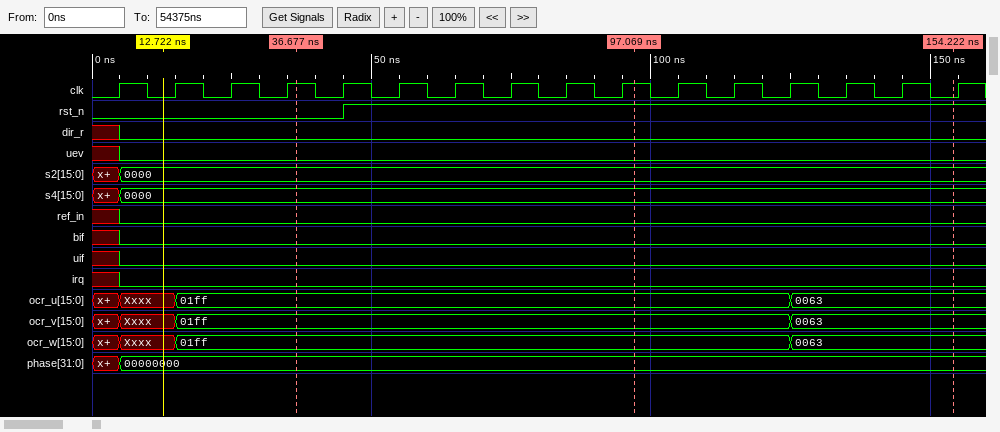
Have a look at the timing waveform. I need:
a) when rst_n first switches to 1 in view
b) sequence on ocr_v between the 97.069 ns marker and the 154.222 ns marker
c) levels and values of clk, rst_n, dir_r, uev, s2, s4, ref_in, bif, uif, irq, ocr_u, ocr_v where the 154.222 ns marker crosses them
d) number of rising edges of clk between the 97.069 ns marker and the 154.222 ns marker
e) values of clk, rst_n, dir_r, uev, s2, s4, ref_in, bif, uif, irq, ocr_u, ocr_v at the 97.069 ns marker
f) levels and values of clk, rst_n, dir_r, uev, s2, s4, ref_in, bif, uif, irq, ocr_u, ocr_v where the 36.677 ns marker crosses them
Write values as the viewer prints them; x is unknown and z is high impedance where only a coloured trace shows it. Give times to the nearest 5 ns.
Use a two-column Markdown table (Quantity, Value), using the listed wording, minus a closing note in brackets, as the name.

| Quantity | Value |
|---|---|
| when rst_n first switches to 1 in view | 45 ns |
| sequence on ocr_v between the 97.069 ns marker and the 154.222 ns marker | 01ff, 0063 |
| levels and values of clk, rst_n, dir_r, uev, s2, s4, ref_in, bif, uif, irq, ocr_u, ocr_v where the 154.222 ns marker crosses them | clk=0, rst_n=1, dir_r=0, uev=0, s2=0000, s4=0000, ref_in=0, bif=0, uif=0, irq=0, ocr_u=0063, ocr_v=0063 |
| number of rising edges of clk between the 97.069 ns marker and the 154.222 ns marker | 5 |
| values of clk, rst_n, dir_r, uev, s2, s4, ref_in, bif, uif, irq, ocr_u, ocr_v at the 97.069 ns marker | clk=1, rst_n=1, dir_r=0, uev=0, s2=0000, s4=0000, ref_in=0, bif=0, uif=0, irq=0, ocr_u=01ff, ocr_v=01ff |
| levels and values of clk, rst_n, dir_r, uev, s2, s4, ref_in, bif, uif, irq, ocr_u, ocr_v where the 36.677 ns marker crosses them | clk=1, rst_n=0, dir_r=0, uev=0, s2=0000, s4=0000, ref_in=0, bif=0, uif=0, irq=0, ocr_u=01ff, ocr_v=01ff |
